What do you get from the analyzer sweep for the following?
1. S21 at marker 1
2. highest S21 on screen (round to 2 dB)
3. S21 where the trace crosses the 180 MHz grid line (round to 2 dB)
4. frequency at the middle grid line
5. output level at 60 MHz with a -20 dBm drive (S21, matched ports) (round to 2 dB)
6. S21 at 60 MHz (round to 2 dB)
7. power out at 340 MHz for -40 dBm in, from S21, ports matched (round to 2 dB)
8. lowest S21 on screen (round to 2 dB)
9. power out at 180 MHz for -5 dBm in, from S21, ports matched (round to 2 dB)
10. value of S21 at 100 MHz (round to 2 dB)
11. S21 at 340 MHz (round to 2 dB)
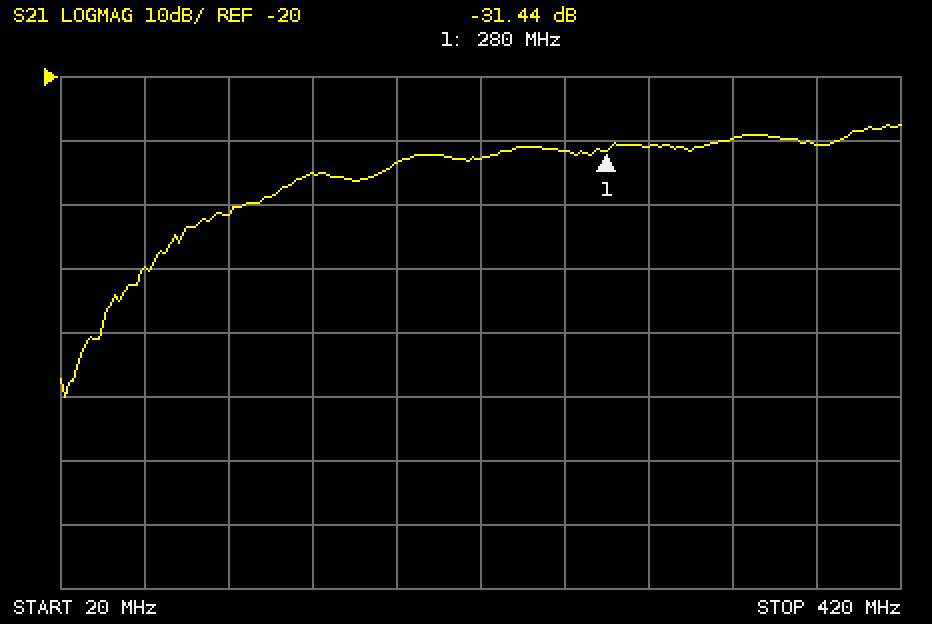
-31.44 dB
-28 dB
-34 dB
220 MHz
-70 dBm
-50 dB
-70 dBm
-70 dB
-38 dBm
-42 dB
-30 dB
